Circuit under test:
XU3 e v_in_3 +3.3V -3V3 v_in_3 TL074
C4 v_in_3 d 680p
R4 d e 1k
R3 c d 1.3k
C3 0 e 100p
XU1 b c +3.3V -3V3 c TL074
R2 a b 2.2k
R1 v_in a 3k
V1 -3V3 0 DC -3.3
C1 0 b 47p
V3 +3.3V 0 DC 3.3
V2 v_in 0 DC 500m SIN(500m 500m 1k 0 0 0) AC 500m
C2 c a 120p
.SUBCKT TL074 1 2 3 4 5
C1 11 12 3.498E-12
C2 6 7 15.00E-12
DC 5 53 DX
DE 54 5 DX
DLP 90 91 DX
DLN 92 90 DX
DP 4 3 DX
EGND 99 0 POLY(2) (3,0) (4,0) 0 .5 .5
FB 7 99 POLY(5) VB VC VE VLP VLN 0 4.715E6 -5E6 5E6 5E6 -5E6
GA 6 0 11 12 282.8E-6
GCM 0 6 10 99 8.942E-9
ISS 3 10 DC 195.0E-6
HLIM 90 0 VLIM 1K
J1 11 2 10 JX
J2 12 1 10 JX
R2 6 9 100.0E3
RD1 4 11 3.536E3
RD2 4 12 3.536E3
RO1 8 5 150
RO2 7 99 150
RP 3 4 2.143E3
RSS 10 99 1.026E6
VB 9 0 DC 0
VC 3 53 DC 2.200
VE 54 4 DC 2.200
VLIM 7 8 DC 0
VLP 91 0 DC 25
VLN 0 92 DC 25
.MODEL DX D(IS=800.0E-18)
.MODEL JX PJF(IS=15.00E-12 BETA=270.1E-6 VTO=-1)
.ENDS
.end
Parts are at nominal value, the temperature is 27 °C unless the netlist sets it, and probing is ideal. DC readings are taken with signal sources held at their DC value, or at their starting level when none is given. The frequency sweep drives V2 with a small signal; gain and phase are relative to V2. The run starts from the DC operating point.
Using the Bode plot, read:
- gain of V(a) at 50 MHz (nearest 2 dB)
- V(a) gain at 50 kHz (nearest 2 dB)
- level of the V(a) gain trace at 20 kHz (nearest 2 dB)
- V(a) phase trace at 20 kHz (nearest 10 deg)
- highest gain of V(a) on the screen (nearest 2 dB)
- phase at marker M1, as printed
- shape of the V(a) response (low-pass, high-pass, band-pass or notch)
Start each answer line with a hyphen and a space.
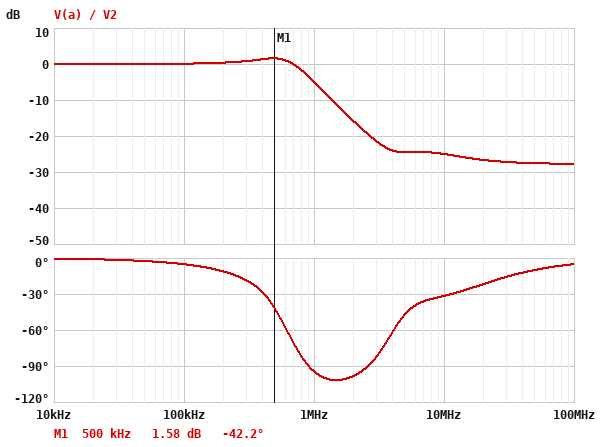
- -28 dB
- 0 dB
- 0 dB
- 0 deg
- 2 dB
- -42.2 deg
- low-pass
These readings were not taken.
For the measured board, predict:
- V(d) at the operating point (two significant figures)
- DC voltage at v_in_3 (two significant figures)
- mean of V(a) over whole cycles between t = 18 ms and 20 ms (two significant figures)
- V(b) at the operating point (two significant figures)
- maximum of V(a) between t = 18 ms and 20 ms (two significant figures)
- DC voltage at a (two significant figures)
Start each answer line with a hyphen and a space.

- 500 mV
- 500 mV
- 500 mV
- 500 mV
- 1.0 V
- 500 mV
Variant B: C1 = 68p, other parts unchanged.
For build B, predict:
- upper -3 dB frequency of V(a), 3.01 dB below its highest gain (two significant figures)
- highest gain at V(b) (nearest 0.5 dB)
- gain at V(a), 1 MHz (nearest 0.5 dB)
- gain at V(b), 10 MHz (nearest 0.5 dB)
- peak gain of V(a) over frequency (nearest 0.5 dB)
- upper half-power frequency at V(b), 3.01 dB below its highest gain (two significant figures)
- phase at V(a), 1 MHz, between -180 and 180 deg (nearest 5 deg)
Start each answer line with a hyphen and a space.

- 690 kHz
- 0 dB
- -7.0 dB
- -44.5 dB
- 0.5 dB
- 620 kHz
- -85 deg
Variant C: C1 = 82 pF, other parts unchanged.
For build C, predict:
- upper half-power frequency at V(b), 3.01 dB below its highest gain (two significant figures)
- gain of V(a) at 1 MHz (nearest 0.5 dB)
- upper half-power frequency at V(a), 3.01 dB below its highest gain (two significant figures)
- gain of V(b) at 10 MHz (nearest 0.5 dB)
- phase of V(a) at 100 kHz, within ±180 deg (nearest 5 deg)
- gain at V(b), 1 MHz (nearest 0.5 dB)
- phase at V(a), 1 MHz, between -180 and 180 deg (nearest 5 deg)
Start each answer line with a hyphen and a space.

- 530 kHz
- -8.0 dB
- 630 kHz
- -46.0 dB
- -10 deg
- -11.5 dB
- -80 deg
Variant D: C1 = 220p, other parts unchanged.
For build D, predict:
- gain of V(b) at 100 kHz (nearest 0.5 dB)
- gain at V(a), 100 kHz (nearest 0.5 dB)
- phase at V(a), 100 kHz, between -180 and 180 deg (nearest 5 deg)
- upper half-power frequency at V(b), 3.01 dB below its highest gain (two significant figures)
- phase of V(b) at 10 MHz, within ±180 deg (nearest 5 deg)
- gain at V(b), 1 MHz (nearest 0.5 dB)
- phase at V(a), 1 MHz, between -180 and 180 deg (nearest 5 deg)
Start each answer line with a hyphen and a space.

- -1.5 dB
- -1.0 dB
- -20 deg
- 160 kHz
- -120 deg
- -20.0 dB
- -60 deg
